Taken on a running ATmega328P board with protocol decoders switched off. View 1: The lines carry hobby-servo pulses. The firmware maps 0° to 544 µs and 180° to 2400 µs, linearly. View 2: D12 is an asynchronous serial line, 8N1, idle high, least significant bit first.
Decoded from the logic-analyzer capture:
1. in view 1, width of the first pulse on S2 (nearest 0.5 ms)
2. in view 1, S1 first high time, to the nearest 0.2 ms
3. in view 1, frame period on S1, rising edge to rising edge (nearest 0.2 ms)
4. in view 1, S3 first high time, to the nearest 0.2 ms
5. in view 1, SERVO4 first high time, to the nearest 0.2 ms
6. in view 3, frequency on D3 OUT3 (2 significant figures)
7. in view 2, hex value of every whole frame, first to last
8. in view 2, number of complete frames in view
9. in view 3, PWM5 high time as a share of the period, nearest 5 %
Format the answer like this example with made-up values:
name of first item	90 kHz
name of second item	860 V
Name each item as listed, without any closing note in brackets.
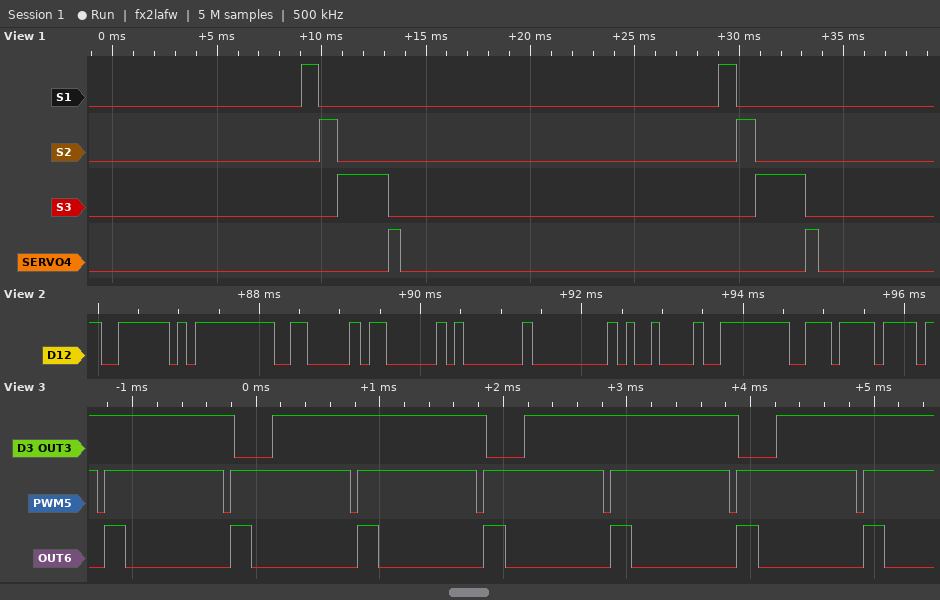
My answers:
in view 1, width of the first pulse on S2	1.0 ms
in view 1, S1 first high time, to the nearest 0.2 ms	0.8 ms
in view 1, frame period on S1, rising edge to rising edge	20.0 ms
in view 1, S3 first high time, to the nearest 0.2 ms	2.4 ms
in view 1, SERVO4 first high time, to the nearest 0.2 ms	0.6 ms
in view 3, frequency on D3 OUT3	490 Hz
in view 2, hex value of every whole frame, first to last	0x7E 0xFF 0x06 0x03 0x01 0x00 0x09 0xFE 0xEE
in view 2, number of complete frames in view	9
in view 3, PWM5 high time as a share of the period, nearest 5 %	95 %
